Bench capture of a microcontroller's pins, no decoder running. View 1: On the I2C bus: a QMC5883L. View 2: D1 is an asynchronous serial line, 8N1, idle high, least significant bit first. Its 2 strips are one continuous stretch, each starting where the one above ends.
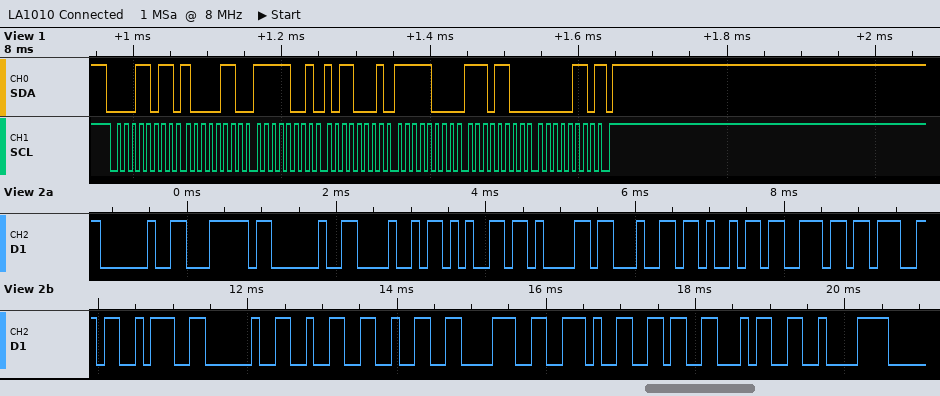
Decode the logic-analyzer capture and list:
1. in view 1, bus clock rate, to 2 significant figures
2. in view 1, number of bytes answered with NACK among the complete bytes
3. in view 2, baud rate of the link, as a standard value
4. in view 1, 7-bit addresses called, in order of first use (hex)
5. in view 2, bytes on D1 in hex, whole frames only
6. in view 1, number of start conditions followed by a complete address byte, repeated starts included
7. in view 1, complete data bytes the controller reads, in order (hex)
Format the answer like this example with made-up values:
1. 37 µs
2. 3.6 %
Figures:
1. 100 kHz
2. 1
3. 9600 baud
4. 0x0D
5. 20 7C 20 48 65 61 64 69 6E 67 3A 20 32 32 38 2E 36 34 C2
6. 1
7. 86 F9 B1 F8 EC 06
